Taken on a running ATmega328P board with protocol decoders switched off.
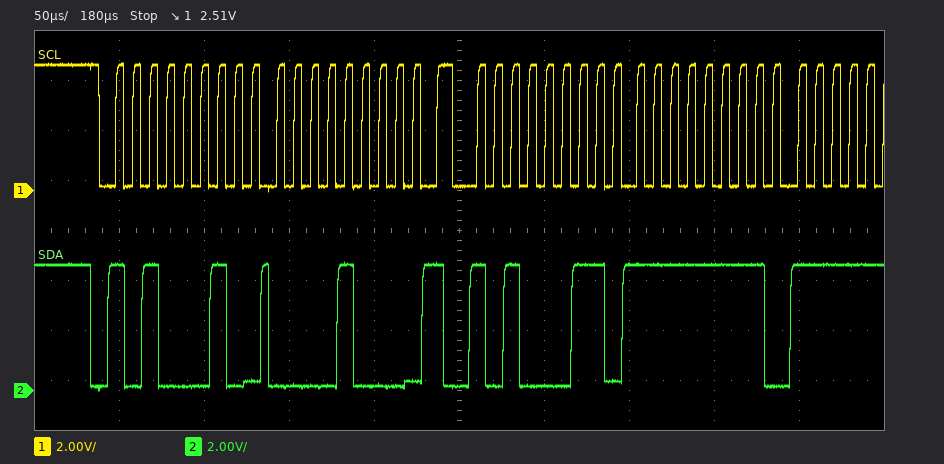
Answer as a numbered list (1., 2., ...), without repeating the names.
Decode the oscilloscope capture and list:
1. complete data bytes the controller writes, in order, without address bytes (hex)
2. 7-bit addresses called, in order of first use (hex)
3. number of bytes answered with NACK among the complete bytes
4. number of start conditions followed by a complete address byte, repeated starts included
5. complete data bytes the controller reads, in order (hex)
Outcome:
1. 08
2. 0x51
3. 0
4. 2
5. FF
